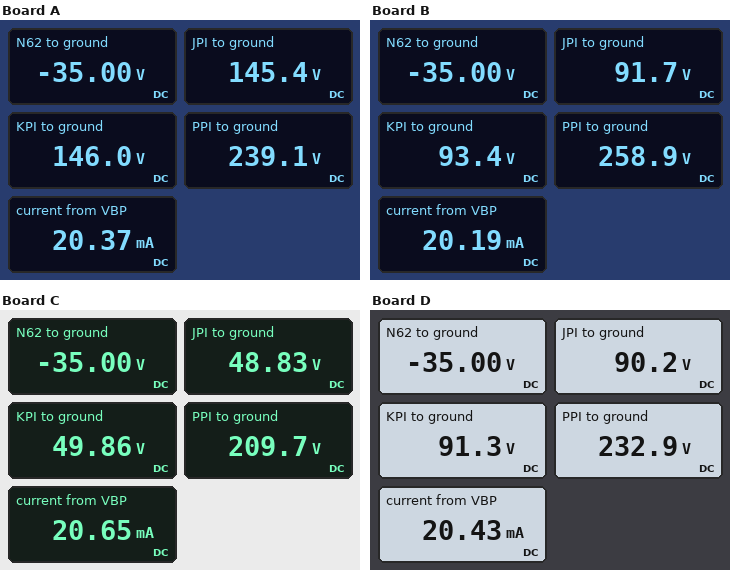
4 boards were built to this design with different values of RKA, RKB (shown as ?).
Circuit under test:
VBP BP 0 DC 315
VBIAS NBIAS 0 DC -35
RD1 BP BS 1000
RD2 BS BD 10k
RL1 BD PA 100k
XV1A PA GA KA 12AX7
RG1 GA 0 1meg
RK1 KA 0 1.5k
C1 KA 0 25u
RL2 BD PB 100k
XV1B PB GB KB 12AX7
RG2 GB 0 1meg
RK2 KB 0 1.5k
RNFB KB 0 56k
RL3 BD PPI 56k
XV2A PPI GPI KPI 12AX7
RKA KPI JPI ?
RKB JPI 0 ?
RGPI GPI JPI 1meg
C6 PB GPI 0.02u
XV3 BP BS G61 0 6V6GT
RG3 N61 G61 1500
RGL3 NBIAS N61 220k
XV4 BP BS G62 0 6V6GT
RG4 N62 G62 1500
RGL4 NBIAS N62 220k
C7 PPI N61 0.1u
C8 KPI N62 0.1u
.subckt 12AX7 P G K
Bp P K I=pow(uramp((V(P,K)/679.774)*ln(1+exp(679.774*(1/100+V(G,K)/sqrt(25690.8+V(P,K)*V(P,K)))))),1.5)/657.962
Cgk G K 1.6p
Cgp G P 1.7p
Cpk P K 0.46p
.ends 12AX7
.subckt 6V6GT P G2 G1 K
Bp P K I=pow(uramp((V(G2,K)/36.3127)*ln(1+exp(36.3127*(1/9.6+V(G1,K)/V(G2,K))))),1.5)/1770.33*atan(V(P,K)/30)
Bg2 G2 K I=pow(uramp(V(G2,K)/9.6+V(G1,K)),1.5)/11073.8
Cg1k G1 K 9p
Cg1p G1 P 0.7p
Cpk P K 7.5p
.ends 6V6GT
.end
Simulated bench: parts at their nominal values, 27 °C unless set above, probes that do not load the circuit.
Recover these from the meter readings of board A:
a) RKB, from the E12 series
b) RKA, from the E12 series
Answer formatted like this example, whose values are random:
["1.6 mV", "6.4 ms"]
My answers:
["180 kΩ", "680 Ω"]
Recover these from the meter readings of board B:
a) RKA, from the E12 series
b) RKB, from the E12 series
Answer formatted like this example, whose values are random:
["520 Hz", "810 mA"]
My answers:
["3.3 kΩ", "180 kΩ"]
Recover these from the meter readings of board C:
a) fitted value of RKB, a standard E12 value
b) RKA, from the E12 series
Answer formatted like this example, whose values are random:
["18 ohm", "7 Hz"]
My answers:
["39 kΩ", "820 Ω"]
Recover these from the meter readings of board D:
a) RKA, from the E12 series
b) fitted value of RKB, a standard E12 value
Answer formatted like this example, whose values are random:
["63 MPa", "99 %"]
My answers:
["1.2 kΩ", "100 kΩ"]
